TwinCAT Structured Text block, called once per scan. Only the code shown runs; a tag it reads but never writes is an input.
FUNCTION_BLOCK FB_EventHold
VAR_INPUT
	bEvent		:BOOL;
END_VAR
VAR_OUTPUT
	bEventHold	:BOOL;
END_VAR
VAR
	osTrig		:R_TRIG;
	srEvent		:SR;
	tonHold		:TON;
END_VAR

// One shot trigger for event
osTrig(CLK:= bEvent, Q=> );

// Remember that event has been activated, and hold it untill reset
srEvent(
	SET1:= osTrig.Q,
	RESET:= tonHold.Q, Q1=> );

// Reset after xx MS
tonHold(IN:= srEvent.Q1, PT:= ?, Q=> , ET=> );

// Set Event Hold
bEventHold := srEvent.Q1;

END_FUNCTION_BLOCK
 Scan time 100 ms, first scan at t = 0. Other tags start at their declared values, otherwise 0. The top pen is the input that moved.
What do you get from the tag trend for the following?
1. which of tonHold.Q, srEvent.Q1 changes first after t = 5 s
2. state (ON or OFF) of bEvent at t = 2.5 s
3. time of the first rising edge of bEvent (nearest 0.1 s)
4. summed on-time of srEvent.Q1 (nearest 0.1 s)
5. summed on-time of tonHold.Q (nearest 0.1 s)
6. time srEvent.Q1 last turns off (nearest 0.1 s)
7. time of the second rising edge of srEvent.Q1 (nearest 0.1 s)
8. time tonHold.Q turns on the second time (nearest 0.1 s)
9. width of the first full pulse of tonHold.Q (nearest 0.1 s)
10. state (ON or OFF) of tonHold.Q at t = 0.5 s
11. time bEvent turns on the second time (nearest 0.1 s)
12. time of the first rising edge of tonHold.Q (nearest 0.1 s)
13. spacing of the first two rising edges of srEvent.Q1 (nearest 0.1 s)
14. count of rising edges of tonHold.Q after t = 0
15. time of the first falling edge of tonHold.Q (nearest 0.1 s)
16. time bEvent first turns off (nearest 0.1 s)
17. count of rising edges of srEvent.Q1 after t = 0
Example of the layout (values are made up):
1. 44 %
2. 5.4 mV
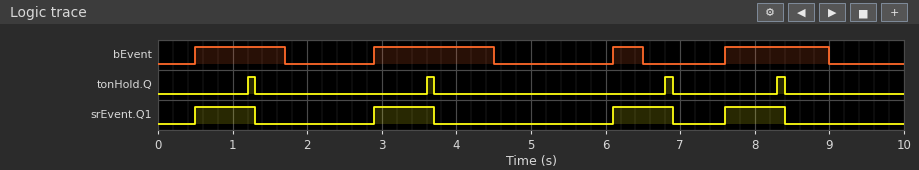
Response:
1. srEvent.Q1
2. OFF
3. 0.5 s
4. 3.2 s
5. 0.4 s
6. 8.4 s
7. 2.9 s
8. 3.6 s
9. 0.1 s
10. OFF
11. 2.9 s
12. 1.2 s
13. 2.4 s
14. 4
15. 1.3 s
16. 1.7 s
17. 4
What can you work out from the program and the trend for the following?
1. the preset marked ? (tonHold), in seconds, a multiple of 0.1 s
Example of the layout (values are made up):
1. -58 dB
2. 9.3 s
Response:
1. 0.7 s
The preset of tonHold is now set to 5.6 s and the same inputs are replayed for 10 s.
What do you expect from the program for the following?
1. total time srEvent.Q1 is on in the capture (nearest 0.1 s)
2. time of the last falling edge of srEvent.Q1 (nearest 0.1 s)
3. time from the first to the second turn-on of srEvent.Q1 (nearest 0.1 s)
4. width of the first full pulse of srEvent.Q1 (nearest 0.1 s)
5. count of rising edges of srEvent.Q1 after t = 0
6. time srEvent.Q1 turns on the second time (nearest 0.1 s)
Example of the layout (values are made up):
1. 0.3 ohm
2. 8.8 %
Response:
1. 8.1 s
2. 6.2 s
3. 7.1 s
4. 5.7 s
5. 2
6. 7.6 s
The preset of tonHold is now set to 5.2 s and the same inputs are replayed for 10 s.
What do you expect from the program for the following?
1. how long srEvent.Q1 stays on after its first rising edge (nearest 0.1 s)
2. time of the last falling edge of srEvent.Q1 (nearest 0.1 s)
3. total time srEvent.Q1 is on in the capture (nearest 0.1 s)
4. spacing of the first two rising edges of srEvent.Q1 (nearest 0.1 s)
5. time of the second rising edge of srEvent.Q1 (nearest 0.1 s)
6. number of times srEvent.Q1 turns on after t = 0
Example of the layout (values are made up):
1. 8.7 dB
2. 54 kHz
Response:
1. 5.3 s
2. 5.8 s
3. 9.2 s
4. 5.6 s
5. 6.1 s
6. 2
